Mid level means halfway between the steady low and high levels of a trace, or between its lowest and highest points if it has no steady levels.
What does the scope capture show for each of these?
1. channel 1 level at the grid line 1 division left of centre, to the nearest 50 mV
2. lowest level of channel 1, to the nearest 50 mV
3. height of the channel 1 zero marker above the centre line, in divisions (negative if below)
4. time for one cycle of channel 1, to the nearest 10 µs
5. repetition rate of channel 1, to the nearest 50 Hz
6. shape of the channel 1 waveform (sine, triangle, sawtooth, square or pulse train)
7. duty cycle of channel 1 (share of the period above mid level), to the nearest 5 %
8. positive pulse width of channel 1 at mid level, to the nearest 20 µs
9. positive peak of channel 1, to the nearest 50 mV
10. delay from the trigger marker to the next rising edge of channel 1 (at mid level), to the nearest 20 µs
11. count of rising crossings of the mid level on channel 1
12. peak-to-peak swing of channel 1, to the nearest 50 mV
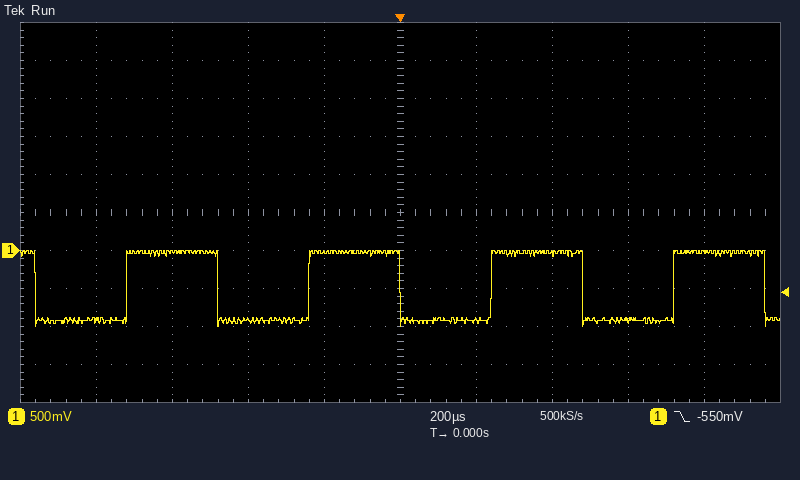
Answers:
0 mV
-1.00 V
-1.0 div
480 µs
2.10 kHz
square
50 %
240 µs
0 mV
240 µs
4
1.00 V
